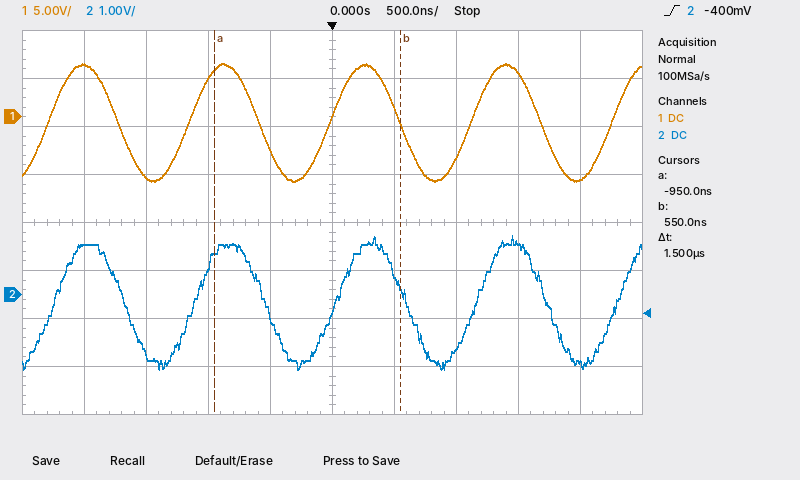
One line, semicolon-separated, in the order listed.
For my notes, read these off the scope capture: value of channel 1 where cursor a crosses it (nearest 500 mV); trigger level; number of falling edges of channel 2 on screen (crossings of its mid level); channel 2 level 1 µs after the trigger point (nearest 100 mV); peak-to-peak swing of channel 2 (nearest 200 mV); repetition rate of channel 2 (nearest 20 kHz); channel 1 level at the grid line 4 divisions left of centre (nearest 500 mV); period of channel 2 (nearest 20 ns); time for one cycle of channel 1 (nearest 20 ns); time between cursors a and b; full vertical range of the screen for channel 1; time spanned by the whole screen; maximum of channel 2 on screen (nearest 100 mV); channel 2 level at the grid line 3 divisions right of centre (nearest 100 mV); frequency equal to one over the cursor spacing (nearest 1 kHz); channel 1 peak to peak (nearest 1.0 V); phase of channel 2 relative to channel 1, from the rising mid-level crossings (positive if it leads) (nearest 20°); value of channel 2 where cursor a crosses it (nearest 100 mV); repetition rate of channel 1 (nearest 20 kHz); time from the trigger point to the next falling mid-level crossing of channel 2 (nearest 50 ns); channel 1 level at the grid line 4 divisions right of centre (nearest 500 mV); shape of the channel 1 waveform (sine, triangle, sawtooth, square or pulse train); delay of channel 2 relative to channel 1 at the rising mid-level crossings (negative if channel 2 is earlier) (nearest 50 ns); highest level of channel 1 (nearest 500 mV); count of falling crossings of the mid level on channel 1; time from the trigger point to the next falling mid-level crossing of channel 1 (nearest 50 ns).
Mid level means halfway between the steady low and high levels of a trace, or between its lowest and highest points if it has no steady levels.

5.0 V; -400 mV; 4; -1.1 V; 2.8 V; 880 kHz; 5.5 V; 1.14 µs; 1.14 µs; 1.5 µs; 40 V; 5 µs; 1.2 V; 1.0 V; 667 kHz; 12.0 V; -20°; 900 mV; 880 kHz; 600 ns; -6.5 V; sine; +50 ns; 5.5 V; 4; 550 ns
